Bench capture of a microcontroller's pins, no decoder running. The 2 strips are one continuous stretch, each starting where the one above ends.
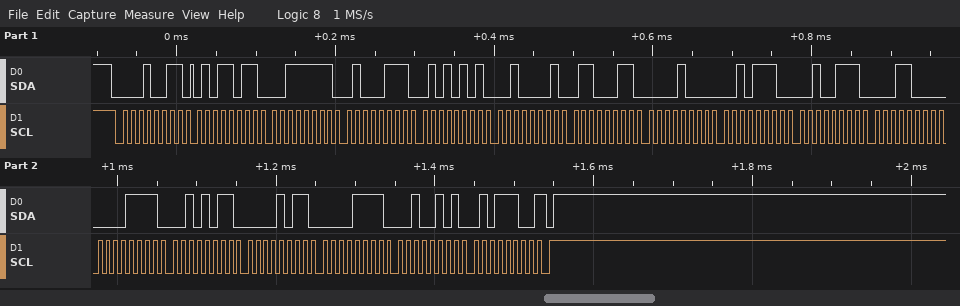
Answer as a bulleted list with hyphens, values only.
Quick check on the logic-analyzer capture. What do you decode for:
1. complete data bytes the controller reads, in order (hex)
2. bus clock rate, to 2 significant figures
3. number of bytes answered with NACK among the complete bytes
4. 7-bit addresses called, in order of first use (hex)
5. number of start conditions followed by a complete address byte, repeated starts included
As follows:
- 5B 3F 47 55 21 63 08 2E 27 18 0F 2B 0B 0F 25 5C
- 100 kHz
- 1
- 0x09
- 1
